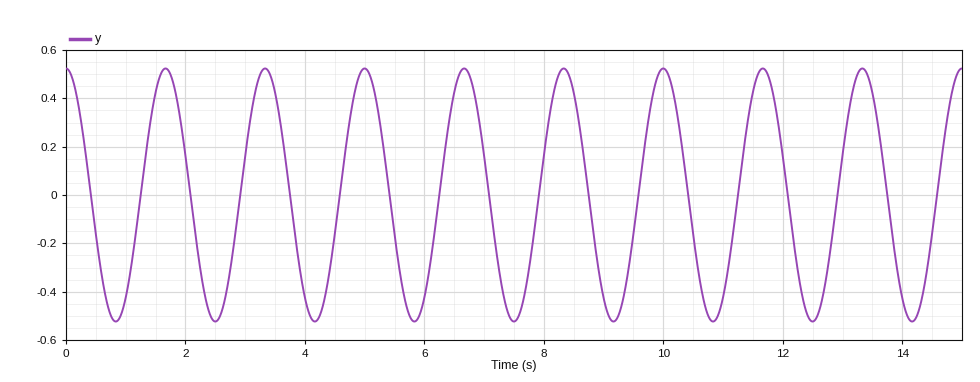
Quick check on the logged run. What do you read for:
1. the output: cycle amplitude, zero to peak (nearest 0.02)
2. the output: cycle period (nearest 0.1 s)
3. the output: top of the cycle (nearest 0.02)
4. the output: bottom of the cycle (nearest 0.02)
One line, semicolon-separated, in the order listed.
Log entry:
0.52; 1.7 s; 0.52; -0.52
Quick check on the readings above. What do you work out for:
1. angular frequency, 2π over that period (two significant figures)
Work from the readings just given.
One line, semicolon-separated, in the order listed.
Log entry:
3.7 rad/s
